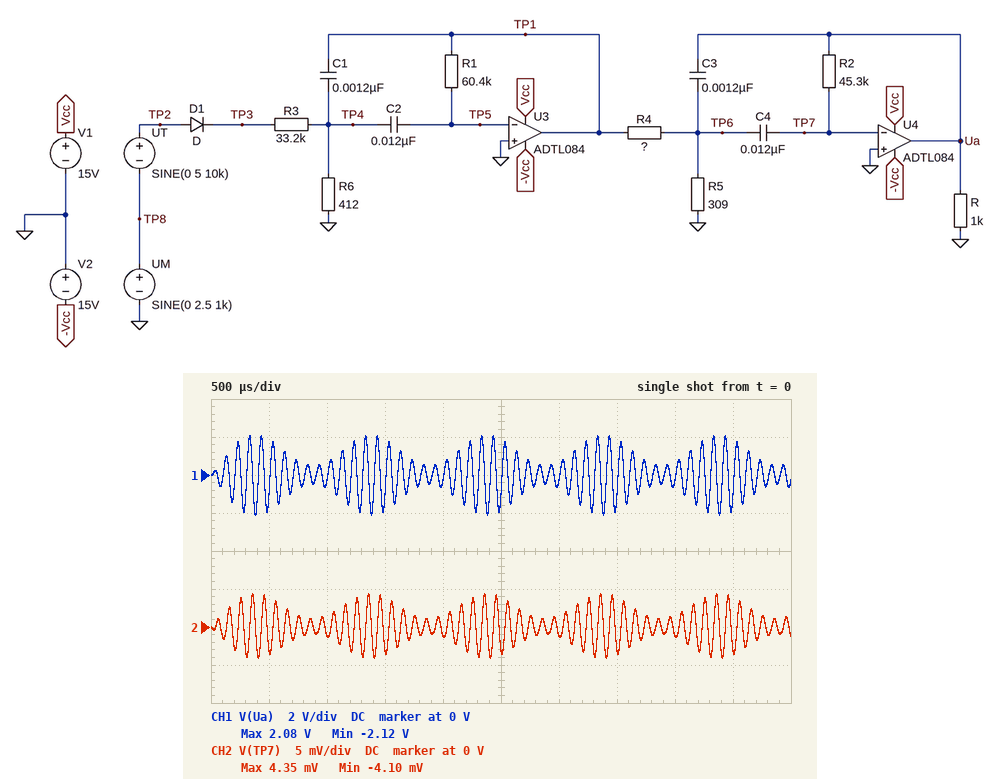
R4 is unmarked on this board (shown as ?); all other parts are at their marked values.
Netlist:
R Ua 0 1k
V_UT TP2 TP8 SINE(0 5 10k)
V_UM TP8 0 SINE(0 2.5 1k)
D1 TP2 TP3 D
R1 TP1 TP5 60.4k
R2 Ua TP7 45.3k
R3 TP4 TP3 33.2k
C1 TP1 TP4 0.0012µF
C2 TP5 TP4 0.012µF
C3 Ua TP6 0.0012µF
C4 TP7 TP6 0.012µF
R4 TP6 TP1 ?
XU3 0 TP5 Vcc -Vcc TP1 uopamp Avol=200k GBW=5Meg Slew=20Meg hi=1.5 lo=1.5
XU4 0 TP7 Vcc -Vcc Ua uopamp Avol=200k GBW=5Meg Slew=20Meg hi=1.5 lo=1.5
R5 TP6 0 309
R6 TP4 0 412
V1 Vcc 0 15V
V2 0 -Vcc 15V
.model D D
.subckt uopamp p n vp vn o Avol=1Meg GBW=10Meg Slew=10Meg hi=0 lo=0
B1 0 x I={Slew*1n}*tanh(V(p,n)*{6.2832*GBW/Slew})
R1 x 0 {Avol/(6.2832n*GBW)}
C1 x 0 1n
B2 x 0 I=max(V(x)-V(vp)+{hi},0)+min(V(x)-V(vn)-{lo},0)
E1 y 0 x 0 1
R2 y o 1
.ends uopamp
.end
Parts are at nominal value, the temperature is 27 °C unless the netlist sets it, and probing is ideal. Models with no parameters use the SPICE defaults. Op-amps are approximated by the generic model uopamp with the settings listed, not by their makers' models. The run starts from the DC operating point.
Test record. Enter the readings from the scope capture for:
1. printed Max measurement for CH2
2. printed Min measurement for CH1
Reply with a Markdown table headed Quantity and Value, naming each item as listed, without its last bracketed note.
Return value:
| Quantity | Value |
|---|---|
| printed Max measurement for CH2 | 4.35 mV |
| printed Min measurement for CH1 | -2.12 V |
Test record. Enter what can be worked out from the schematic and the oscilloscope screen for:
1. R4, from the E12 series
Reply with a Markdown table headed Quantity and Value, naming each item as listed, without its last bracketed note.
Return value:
| Quantity | Value |
|---|---|
| R4, from the E12 series | 56 kΩ |
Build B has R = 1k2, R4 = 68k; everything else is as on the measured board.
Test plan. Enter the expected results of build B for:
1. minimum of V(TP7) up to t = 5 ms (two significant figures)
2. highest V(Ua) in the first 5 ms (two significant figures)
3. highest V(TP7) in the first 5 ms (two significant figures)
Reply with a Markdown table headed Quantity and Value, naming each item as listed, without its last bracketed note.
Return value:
| Quantity | Value |
|---|---|
| minimum of V(TP7) up to t = 5 ms | -3.4 mV |
| highest V(Ua) in the first 5 ms | 1.7 V |
| highest V(TP7) in the first 5 ms | 3.6 mV |
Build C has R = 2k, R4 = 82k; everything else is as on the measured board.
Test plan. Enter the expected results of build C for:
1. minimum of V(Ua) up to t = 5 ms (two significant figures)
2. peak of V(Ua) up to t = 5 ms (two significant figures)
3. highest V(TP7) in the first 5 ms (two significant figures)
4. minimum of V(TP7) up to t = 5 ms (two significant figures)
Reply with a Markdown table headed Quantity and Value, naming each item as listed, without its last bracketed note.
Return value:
| Quantity | Value |
|---|---|
| minimum of V(Ua) up to t = 5 ms | -1.5 V |
| peak of V(Ua) up to t = 5 ms | 1.4 V |
| highest V(TP7) in the first 5 ms | 3.0 mV |
| minimum of V(TP7) up to t = 5 ms | -2.8 mV |
